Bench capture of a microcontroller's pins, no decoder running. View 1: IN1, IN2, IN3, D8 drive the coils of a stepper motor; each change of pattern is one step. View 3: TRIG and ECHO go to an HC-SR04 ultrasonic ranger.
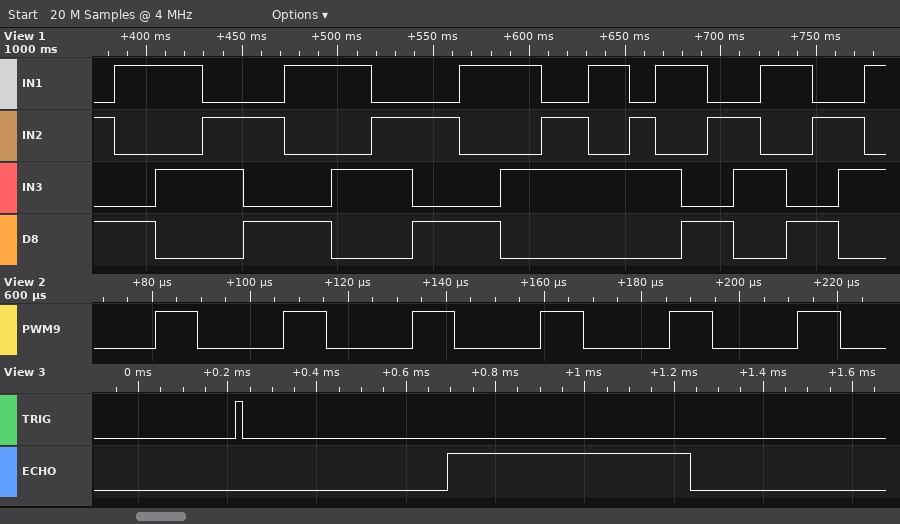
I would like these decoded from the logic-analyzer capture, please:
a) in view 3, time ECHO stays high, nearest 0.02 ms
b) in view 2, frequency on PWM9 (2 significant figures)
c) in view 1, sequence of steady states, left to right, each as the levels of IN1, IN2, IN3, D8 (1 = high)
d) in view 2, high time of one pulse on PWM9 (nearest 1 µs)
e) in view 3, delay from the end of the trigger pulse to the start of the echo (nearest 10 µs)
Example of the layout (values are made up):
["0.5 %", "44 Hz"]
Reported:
["0.54 ms", "38 kHz", "0101 1001 1010 0110 0101 1001 1010 0110 0101 1001 1010 0110 1010 0110 1010 1001 0101 0110 1010 1001 0101 0110 1010", "9 µs", "460 µs"]
